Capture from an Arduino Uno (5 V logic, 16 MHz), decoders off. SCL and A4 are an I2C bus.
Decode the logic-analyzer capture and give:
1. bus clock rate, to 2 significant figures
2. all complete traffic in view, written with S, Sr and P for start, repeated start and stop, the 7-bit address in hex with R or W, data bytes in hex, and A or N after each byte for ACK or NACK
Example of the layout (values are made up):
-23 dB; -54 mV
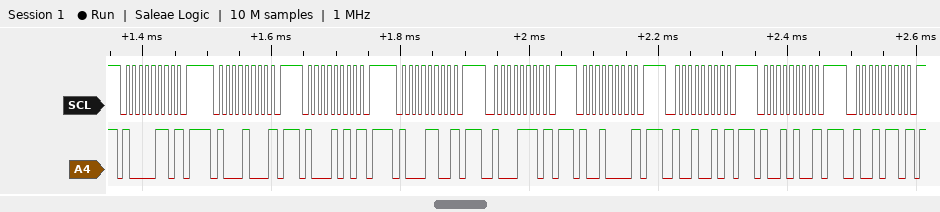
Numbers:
100 kHz; S 43W N P S 44W N P S 45W N P S 46W N P S 47W N P S 48W N P S 49W N P S 4AW N P S 4BW N P
